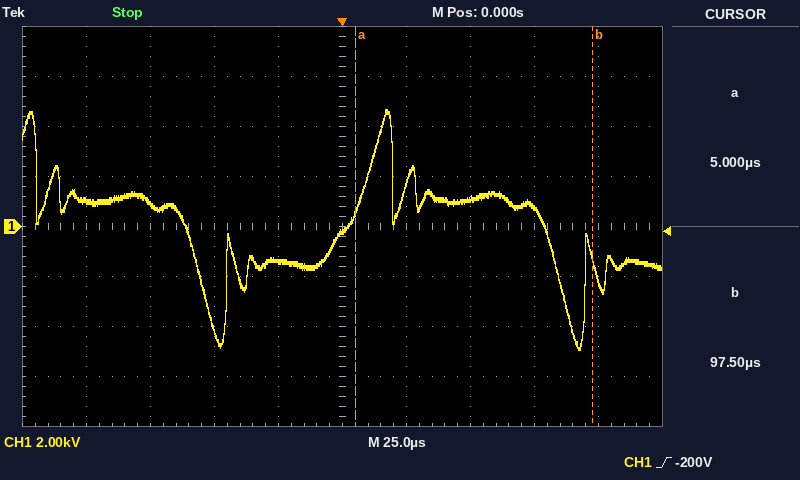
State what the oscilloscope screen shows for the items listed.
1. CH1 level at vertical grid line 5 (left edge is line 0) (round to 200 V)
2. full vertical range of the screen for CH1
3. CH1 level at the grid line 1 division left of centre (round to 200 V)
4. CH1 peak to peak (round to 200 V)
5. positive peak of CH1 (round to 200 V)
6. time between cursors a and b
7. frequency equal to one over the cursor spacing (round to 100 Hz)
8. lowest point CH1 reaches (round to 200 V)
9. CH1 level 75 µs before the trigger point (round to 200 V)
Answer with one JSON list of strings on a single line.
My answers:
["-200 V", "16 kV", "-1.4 kV", "9.6 kV", "4.6 kV", "92.5 µs", "10.8 kHz", "-5.0 kV", "1.0 kV"]
